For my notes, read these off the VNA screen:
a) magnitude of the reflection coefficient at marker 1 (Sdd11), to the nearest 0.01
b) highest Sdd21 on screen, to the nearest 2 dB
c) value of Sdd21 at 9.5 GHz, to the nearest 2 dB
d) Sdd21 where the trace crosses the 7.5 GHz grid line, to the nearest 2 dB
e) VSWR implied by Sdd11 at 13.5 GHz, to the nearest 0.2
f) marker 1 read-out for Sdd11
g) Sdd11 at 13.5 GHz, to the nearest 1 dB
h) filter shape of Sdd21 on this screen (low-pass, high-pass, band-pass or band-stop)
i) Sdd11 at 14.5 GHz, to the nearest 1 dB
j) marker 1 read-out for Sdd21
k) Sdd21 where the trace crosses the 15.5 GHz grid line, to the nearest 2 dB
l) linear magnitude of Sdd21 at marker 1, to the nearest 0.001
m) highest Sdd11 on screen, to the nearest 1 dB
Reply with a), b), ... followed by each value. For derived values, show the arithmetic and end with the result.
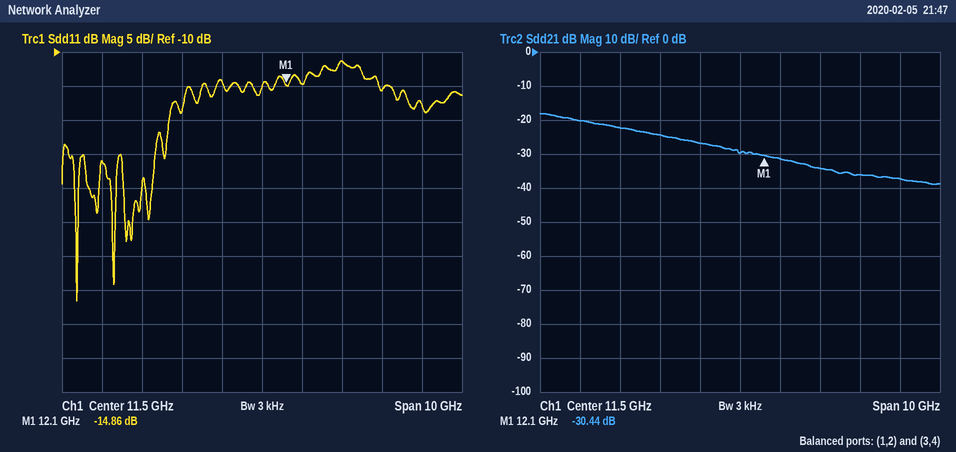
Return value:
a) 10^(-14.86/20) ≈ 0.18
b) -18 dB
c) -24 dB
d) -20 dB
e) |Γ| = 10^(-11/20) = 0.2818; VSWR = (1 + 0.2818)/(1 − 0.2818) ≈ 1.8
f) -14.86 dB
g) -11 dB
h) low-pass
i) -16 dB
j) -30.44 dB
k) -38 dB
l) 10^(-30.44/20) ≈ 0.030
m) -11 dB
